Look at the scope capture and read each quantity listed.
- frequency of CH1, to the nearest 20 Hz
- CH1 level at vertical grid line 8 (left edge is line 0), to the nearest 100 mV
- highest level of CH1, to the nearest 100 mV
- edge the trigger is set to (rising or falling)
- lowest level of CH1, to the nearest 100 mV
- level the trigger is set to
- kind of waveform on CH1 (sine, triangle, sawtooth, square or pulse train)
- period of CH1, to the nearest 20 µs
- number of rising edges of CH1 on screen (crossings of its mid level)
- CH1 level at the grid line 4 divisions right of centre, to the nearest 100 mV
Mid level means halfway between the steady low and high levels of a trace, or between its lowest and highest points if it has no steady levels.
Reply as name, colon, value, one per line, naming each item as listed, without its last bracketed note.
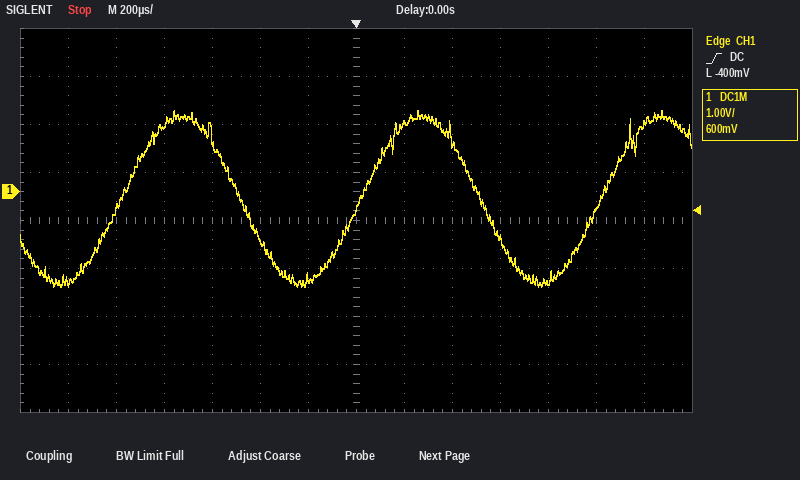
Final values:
frequency of CH1, to the nearest 20 Hz: 1.00 kHz
CH1 level at vertical grid line 8 (left edge is line 0), to the nearest 100 mV: 1.4 V
highest level of CH1, to the nearest 100 mV: 1.7 V
edge the trigger is set to: rising
lowest level of CH1, to the nearest 100 mV: -2.0 V
level the trigger is set to: -400 mV
kind of waveform on CH1: sine
period of CH1, to the nearest 20 µs: 1.00 ms
number of rising edges of CH1 on screen: 3
CH1 level at the grid line 4 divisions right of centre, to the nearest 100 mV: -1.9 V
